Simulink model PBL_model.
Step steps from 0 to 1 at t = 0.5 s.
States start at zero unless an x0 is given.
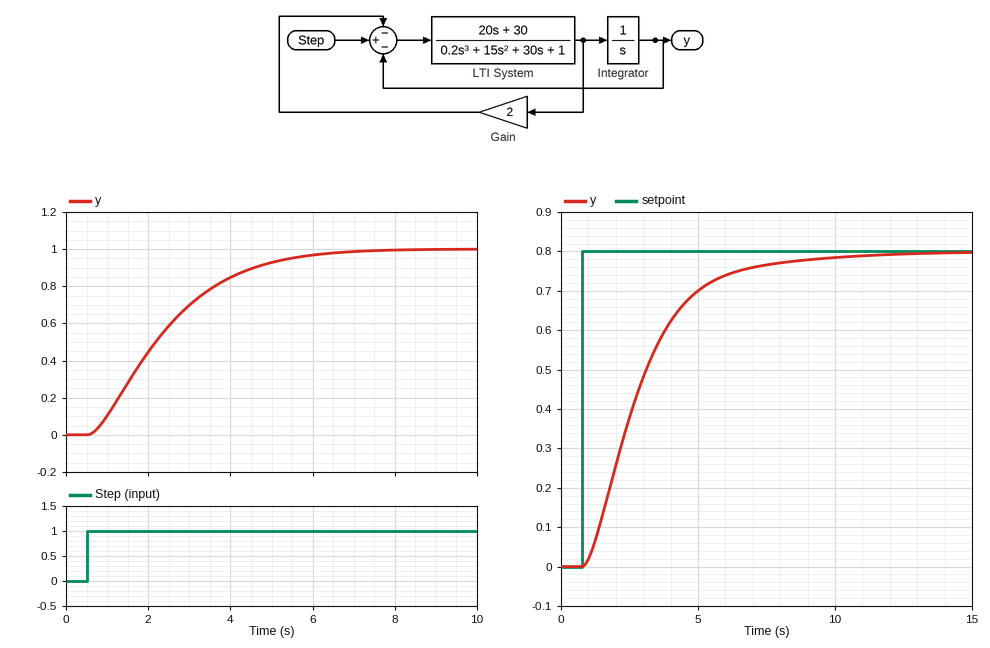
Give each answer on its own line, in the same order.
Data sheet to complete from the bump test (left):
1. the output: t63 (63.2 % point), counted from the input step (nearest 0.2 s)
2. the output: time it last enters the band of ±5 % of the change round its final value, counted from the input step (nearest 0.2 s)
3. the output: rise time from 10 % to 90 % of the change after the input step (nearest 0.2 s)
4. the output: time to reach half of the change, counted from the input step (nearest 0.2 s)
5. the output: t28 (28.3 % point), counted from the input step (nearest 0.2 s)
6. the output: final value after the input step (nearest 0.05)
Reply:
2.2 s
5.0 s
3.6 s
1.6 s
1.0 s
1.00
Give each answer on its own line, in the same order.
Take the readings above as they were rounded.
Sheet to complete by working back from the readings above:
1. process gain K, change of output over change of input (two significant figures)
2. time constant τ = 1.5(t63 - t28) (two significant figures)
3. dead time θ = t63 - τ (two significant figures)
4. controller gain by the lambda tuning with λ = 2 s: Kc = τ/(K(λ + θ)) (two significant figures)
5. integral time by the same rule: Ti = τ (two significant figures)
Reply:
1.0
1.8 s
0.40 s
0.75
1.8 s
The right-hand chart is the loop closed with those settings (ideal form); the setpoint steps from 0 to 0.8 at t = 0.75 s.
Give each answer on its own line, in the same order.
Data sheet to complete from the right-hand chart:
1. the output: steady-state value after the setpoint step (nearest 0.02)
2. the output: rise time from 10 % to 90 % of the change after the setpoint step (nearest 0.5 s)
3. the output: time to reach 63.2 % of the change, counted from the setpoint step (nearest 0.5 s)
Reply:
0.80
4.0 s
2.5 s
